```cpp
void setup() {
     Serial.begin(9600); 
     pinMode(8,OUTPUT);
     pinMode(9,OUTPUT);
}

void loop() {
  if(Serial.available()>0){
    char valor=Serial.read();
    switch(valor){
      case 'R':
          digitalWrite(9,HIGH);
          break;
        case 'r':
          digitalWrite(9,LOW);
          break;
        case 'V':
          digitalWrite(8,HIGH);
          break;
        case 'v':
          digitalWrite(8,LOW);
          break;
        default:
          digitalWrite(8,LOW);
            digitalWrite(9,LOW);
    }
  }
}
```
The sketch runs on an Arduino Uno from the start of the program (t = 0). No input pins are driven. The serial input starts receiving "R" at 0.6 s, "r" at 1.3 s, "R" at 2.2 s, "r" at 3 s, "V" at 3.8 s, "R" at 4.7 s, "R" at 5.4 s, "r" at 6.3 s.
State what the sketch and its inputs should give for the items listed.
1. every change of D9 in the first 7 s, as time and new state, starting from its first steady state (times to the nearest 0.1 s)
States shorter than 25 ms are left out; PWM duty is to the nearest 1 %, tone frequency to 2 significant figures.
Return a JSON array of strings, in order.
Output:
["0 s low; 0.6 s high; 1.3 s low; 2.2 s high; 3 s low; 4.7 s high; 6.3 s low"]
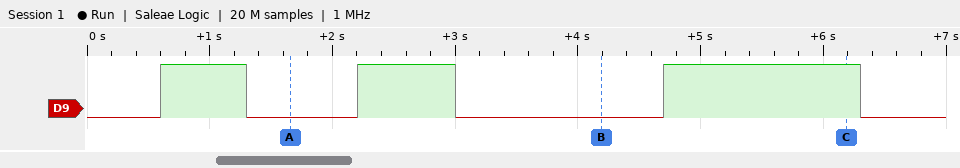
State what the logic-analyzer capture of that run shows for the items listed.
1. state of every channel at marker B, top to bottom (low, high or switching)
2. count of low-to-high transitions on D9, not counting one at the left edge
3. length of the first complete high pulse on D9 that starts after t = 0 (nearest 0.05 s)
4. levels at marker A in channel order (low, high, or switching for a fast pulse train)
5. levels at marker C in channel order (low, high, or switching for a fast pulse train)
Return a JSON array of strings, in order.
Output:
["D9 low", "3", "0.70 s", "D9 low", "D9 high"]
